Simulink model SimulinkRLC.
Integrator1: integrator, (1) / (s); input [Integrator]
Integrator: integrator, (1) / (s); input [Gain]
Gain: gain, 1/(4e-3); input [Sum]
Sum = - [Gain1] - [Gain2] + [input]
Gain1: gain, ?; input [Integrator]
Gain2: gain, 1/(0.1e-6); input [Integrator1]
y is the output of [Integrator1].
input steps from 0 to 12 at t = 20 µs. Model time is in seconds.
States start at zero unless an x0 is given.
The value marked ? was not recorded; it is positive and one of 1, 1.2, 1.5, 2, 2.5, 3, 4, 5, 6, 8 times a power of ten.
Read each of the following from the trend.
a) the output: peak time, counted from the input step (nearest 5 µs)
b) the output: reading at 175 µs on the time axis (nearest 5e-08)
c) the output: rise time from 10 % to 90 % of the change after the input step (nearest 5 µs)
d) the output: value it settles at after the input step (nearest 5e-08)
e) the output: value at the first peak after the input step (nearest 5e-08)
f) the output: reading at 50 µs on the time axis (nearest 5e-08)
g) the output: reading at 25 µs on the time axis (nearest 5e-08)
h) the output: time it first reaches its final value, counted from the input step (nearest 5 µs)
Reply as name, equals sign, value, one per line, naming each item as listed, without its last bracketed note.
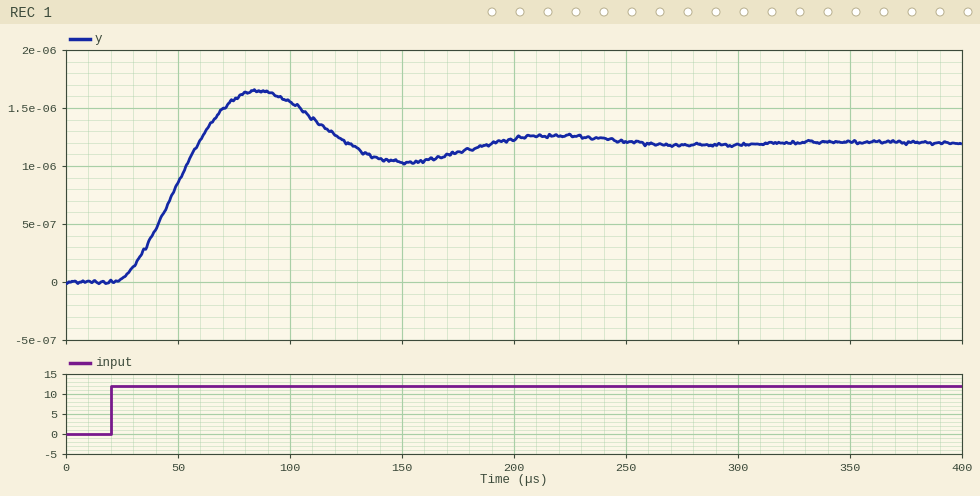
the output: peak time, counted from the input step = 65 µs
the output: reading at 175 µs on the time axis = 0.00000110
the output: rise time from 10 % to 90 % of the change after the input step = 25 µs
the output: value it settles at after the input step = 0.00000120
the output: value at the first peak after the input step = 0.00000165
the output: reading at 50 µs on the time axis = 0.00000085
the output: reading at 25 µs on the time axis = 0.00000005
the output: time it first reaches its final value, counted from the input step = 40 µs
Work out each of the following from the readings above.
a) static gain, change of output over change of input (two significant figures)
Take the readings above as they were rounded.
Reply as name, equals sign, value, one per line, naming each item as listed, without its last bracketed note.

static gain, change of output over change of input = 0.00000010
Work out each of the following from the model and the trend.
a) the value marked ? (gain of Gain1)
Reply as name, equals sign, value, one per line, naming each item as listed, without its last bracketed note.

the value marked ? = 120
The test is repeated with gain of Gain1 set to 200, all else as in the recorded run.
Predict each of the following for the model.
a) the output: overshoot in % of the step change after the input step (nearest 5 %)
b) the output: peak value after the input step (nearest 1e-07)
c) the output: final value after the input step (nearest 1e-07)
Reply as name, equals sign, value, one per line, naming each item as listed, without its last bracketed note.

the output: overshoot in % of the step change after the input step = 15 %
the output: peak value after the input step = 0.0000014
the output: final value after the input step = 0.0000012
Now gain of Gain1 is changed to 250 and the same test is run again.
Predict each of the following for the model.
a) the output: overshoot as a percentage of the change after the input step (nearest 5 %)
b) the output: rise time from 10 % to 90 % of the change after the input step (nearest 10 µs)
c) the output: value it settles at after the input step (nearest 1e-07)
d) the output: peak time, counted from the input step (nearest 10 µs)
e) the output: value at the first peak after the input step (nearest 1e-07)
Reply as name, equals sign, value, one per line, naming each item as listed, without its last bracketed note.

the output: overshoot as a percentage of the change after the input step = 10 %
the output: rise time from 10 % to 90 % of the change after the input step = 40 µs
the output: value it settles at after the input step = 0.0000012
the output: peak time, counted from the input step = 80 µs
the output: value at the first peak after the input step = 0.0000013
